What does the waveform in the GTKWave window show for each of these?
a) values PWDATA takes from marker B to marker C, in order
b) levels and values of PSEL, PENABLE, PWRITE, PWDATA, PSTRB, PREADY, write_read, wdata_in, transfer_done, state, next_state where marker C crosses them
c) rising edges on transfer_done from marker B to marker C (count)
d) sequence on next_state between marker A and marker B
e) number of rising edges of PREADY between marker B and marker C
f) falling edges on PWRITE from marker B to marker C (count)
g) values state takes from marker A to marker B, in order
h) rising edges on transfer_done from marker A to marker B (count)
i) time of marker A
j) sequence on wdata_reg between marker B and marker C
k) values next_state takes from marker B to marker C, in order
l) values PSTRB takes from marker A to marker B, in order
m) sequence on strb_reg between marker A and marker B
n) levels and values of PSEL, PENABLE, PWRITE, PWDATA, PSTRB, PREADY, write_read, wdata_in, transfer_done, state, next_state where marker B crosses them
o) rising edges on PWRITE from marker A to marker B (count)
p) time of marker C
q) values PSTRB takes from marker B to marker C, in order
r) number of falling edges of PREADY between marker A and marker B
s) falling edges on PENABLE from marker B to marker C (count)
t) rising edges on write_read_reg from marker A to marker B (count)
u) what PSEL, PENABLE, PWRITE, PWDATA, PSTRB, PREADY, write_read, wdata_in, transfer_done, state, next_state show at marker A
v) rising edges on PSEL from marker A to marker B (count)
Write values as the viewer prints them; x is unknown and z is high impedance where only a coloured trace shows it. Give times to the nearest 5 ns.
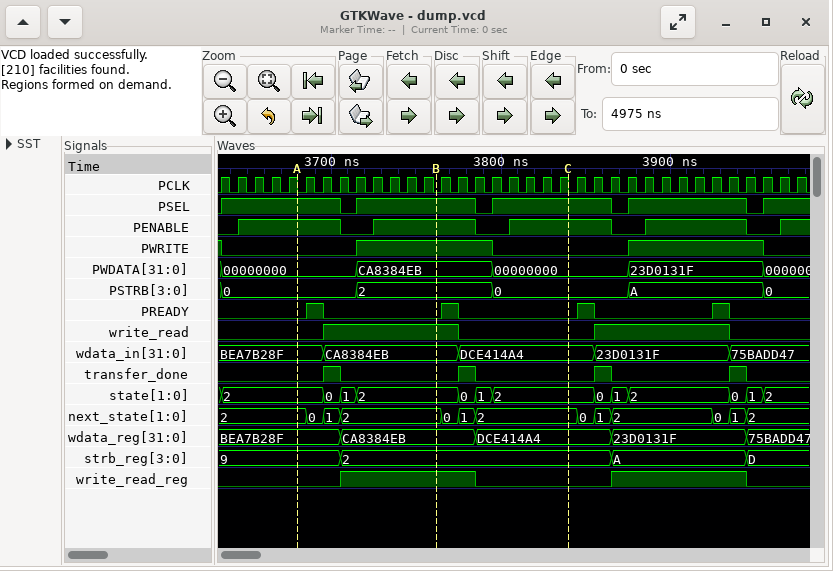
CA8384EB, 00000000
PSEL=1, PENABLE=1, PWRITE=0, PWDATA=00000000, PSTRB=0, PREADY=0, write_read=0, wdata_in=DCE414A4, transfer_done=0, state=2, next_state=2
1
2, 0, 1, 2
1
1
2, 0, 1, 2
1
3680 ns
CA8384EB, DCE414A4
2, 0, 1, 2
0, 2
9, 2
PSEL=1, PENABLE=1, PWRITE=1, PWDATA=CA8384EB, PSTRB=2, PREADY=0, write_read=1, wdata_in=CA8384EB, transfer_done=0, state=2, next_state=2
1
3840 ns
2, 0
1
1
1
PSEL=1, PENABLE=1, PWRITE=0, PWDATA=00000000, PSTRB=0, PREADY=0, write_read=0, wdata_in=BEA7B28F, transfer_done=0, state=2, next_state=2
1
